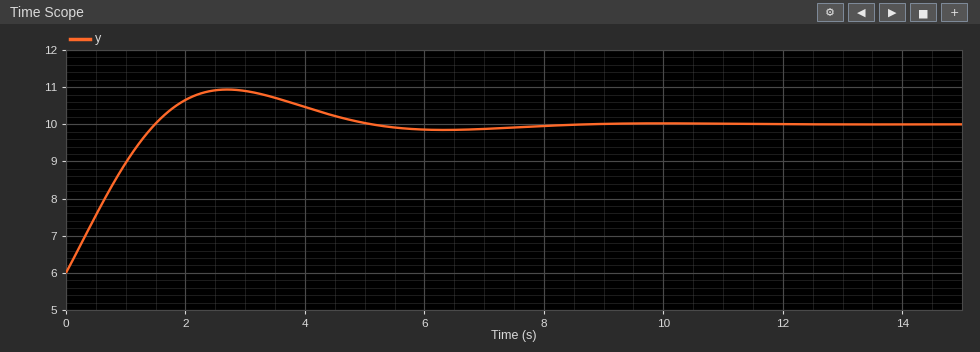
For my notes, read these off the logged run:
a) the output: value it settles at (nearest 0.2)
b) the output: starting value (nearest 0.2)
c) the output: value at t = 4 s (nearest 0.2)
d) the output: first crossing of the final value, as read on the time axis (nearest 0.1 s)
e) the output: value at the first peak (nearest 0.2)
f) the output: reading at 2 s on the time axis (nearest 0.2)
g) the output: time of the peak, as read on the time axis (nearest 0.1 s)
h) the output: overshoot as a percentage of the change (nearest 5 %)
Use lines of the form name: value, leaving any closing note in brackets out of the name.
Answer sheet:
the output: value it settles at: 10.0
the output: starting value: 6.0
the output: value at t = 4 s: 10.4
the output: first crossing of the final value, as read on the time axis: 1.5 s
the output: value at the first peak: 11.0
the output: reading at 2 s on the time axis: 10.6
the output: time of the peak, as read on the time axis: 2.7 s
the output: overshoot as a percentage of the change: 25 %
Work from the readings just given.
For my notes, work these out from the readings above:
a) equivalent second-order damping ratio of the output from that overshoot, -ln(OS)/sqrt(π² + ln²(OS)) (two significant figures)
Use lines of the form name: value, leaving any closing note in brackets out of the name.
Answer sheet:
equivalent second-order damping ratio of the output from that overshoot, -ln(OS)/sqrt(π² + ln²(OS)): 0.40
